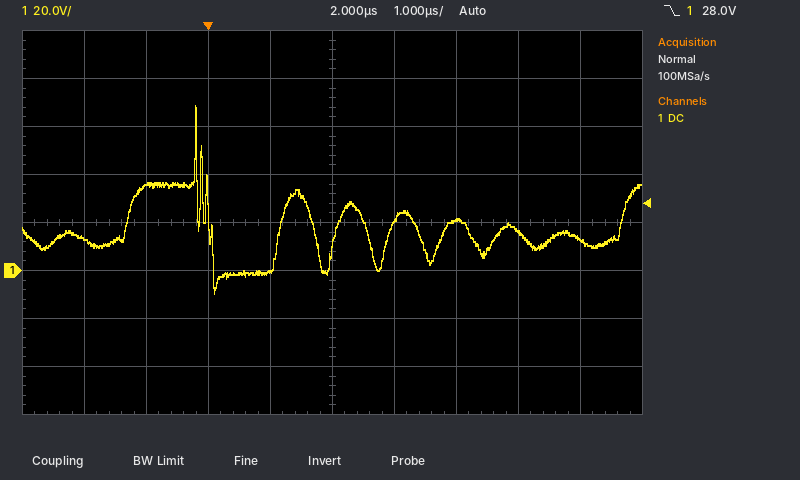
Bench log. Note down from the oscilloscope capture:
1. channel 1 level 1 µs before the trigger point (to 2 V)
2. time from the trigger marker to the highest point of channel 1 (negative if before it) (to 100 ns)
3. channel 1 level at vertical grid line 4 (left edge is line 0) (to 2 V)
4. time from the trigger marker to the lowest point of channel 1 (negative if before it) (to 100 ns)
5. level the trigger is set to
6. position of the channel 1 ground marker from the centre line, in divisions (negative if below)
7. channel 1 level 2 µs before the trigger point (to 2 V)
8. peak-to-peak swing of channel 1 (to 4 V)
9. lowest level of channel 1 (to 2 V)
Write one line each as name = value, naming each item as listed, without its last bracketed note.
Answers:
channel 1 level 1 µs before the trigger point = 36 V
time from the trigger marker to the highest point of channel 1 (negative if before it) = -200 ns
channel 1 level at vertical grid line 4 (left edge is line 0) = 0 V
time from the trigger marker to the lowest point of channel 1 (negative if before it) = +100 ns
level the trigger is set to = 28.0 V
position of the channel 1 ground marker from the centre line, in divisions = -1.0 div
channel 1 level 2 µs before the trigger point = 14 V
peak-to-peak swing of channel 1 = 80 V
lowest level of channel 1 = -10 V
